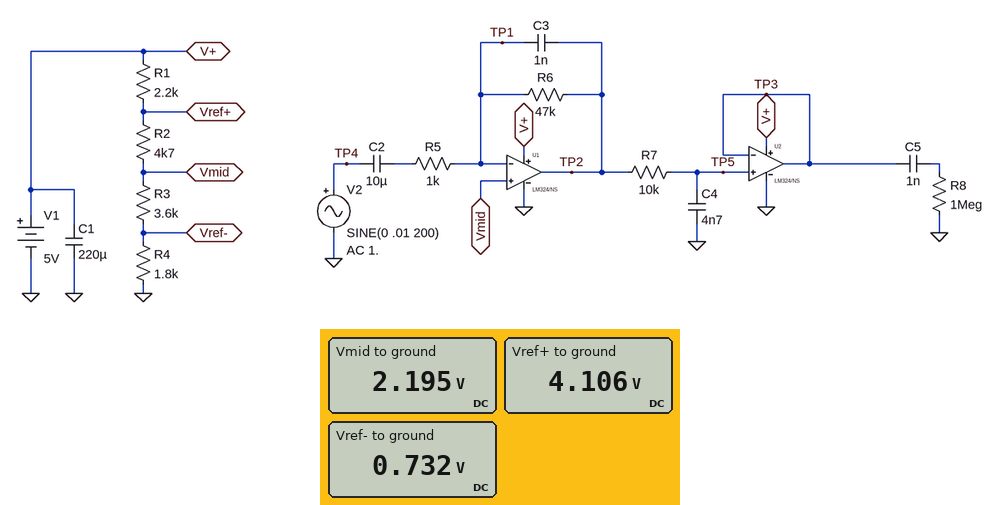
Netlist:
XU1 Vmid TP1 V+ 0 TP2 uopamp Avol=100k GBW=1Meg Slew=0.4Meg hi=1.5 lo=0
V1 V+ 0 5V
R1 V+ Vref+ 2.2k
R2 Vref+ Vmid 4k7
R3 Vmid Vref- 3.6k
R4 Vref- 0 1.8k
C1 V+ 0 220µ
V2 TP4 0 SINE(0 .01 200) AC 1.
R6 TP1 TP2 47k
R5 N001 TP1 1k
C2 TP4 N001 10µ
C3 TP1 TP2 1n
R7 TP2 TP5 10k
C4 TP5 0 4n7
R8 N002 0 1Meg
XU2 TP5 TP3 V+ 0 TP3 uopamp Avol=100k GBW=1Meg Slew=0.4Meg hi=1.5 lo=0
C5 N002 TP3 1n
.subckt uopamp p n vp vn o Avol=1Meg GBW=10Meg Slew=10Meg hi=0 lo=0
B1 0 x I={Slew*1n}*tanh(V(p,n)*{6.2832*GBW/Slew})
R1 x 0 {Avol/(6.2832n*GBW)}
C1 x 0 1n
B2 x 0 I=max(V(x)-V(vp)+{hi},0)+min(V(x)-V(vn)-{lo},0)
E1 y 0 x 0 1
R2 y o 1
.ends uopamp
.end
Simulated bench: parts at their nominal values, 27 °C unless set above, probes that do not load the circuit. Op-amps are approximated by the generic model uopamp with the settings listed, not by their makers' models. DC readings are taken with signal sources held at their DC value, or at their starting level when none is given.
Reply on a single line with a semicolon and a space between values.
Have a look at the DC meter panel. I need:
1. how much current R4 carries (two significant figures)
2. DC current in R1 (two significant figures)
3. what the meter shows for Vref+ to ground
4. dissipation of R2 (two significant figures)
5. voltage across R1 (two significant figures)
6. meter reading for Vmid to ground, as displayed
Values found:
410 µA; 410 µA; 4.106 V; 780 µW; 890 mV; 2.195 V
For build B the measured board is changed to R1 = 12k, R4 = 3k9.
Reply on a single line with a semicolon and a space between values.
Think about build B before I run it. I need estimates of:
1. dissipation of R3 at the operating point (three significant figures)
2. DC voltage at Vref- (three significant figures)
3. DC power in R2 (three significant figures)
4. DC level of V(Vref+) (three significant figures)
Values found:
154 µW; 806 mV; 201 µW; 2.52 V
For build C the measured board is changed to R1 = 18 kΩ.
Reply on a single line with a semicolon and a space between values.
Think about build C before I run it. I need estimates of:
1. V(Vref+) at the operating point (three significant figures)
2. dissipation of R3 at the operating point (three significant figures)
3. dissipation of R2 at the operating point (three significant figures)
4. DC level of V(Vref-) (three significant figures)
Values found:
1.80 V; 114 µW; 149 µW; 320 mV
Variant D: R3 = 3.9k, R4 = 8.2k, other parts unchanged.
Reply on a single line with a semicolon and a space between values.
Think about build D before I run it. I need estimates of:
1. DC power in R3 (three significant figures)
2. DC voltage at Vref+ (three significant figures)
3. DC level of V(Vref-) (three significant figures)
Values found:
270 µW; 4.42 V; 2.16 V
